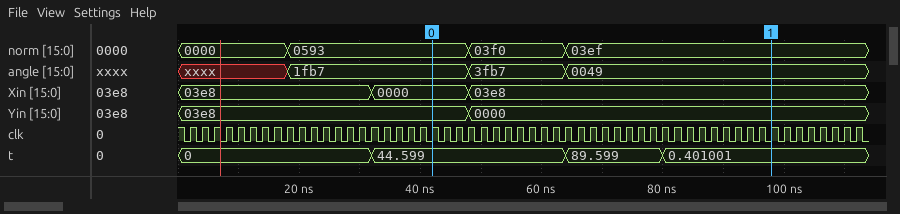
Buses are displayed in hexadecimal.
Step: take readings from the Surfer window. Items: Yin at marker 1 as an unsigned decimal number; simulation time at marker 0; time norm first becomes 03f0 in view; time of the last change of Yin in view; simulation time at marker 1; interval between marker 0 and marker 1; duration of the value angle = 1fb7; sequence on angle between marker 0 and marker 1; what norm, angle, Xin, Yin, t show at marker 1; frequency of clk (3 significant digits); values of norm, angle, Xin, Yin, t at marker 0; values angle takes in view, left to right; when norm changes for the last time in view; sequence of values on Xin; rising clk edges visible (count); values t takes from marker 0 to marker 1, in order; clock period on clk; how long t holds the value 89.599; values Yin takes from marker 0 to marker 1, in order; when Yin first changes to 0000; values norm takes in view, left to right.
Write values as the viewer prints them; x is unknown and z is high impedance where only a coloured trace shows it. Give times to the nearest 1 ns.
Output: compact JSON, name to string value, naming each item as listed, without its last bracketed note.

{"Yin at marker 1 as an unsigned decimal number": "0", "simulation time at marker 0": "42 ns", "time norm first becomes 03f0 in view": "48 ns", "time of the last change of Yin in view": "48 ns", "simulation time at marker 1": "98 ns", "interval between marker 0 and marker 1": "56 ns", "duration of the value angle = 1fb7": "30 ns", "sequence on angle between marker 0 and marker 1": "1fb7, 3fb7, 0049", "what norm, angle, Xin, Yin, t show at marker 1": "norm=03ef, angle=0049, Xin=03e8, Yin=0000, t=0.401001", "frequency of clk": "500 MHz", "values of norm, angle, Xin, Yin, t at marker 0": "norm=0593, angle=1fb7, Xin=0000, Yin=03e8, t=44.599", "values angle takes in view, left to right": "xxxx, 1fb7, 3fb7, 0049", "when norm changes for the last time in view": "64 ns", "sequence of values on Xin": "03e8, 0000, 03e8", "rising clk edges visible": "56", "values t takes from marker 0 to marker 1, in order": "44.599, 89.599, 0.401001", "clock period on clk": "2 ns", "how long t holds the value 89.599": "16 ns", "values Yin takes from marker 0 to marker 1, in order": "03e8, 0000", "when Yin first changes to 0000": "48 ns", "values norm takes in view, left to right": "0000, 0593, 03f0, 03ef"}
